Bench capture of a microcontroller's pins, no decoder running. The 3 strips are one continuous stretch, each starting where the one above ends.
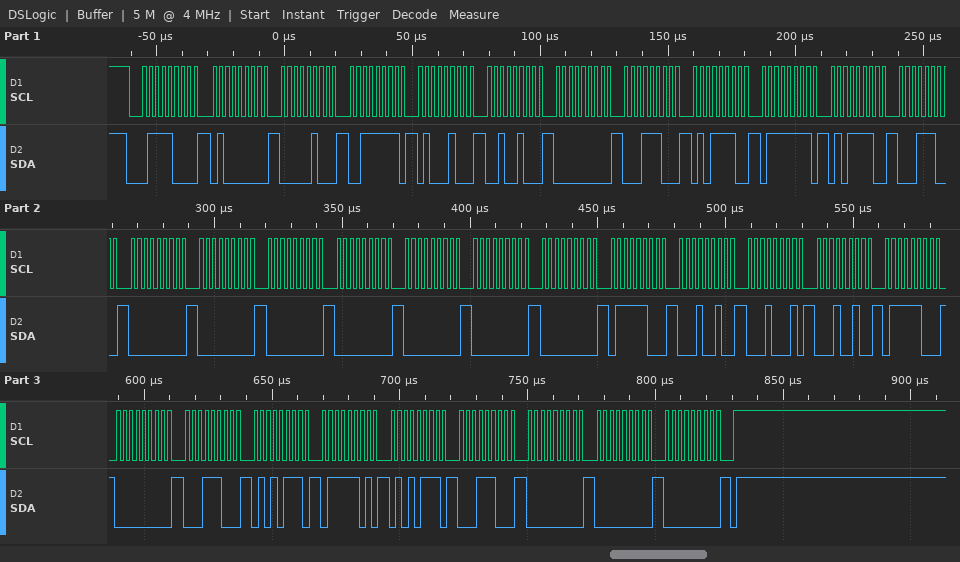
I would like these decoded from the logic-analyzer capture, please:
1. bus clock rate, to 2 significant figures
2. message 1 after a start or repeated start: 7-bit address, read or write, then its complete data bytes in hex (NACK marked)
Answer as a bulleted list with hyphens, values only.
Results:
- 400 kHz
- 0x3C write: 40 04 3F 44 24 00 1C 5E 7F 5E 1C 00 00 00 00 00 00 00 7C 12 11 12 7C 00 1C 57 7D 57 1C 00 00 00
